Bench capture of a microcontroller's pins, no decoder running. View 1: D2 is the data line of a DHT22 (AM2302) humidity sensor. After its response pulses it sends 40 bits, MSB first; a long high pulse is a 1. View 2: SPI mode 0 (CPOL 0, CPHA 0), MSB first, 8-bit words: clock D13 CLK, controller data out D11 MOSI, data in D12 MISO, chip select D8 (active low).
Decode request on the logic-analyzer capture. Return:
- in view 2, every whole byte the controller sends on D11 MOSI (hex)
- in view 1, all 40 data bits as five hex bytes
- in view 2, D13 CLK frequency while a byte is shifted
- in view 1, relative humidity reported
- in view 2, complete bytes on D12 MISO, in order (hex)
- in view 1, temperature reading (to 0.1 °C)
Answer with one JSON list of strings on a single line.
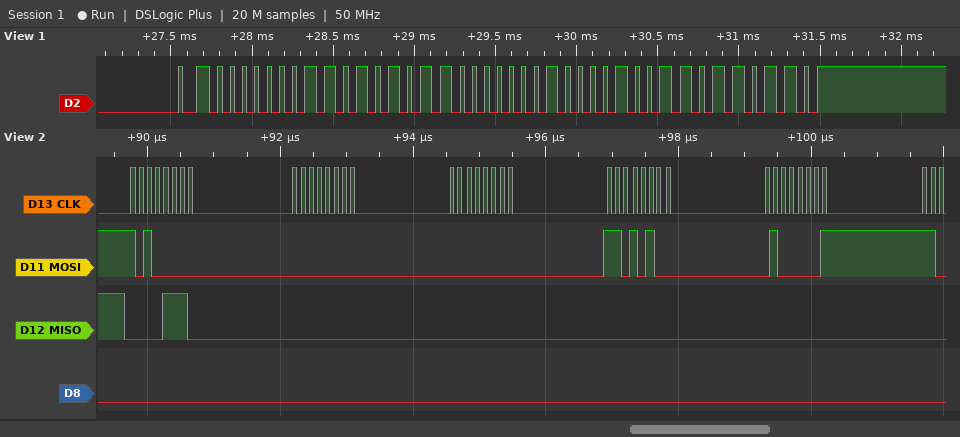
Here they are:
["A0 00 00 D4 41", "01 AB 01 09 B6", "8 MHz", "42.7 %", "0E 00 00 00 00", "26.5 °C"]
